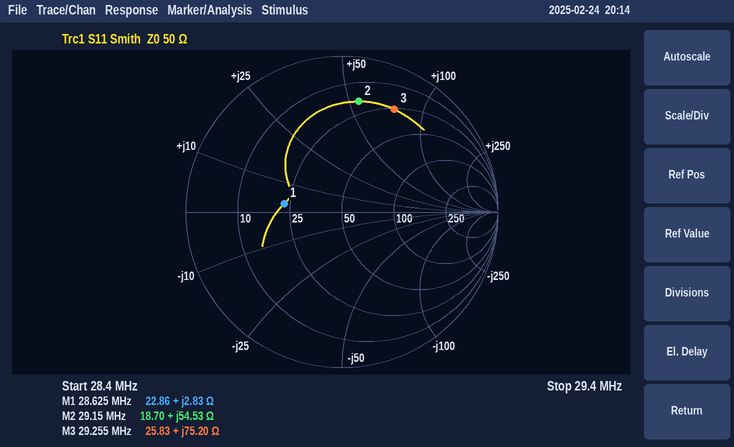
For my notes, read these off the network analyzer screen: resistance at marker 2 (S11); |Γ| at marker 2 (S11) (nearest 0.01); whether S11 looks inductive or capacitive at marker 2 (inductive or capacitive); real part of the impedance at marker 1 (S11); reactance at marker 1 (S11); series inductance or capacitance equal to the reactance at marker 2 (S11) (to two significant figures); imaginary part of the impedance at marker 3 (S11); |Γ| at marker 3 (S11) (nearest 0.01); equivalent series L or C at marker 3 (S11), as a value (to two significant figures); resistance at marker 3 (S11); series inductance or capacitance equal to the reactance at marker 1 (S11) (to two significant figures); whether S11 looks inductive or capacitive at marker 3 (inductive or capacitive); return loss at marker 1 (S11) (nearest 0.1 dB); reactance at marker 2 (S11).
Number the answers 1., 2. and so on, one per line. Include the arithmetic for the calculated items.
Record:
1. 18.70 Ω
2. 0.72
3. inductive
4. 22.86 Ω
5. +2.83 Ω
6. L = 54.53 Ω/(2π × 29.15 MHz) ≈ 298 nH, so 300 nH to two significant figures
7. +75.20 Ω
8. 0.74
9. L = 75.2 Ω/(2π × 29.255 MHz) ≈ 409 nH, so 410 nH to two significant figures
10. 25.83 Ω
11. L = 2.83 Ω/(2π × 28.625 MHz) ≈ 16 nH
12. inductive
13. 8.5 dB
14. +54.53 Ω
